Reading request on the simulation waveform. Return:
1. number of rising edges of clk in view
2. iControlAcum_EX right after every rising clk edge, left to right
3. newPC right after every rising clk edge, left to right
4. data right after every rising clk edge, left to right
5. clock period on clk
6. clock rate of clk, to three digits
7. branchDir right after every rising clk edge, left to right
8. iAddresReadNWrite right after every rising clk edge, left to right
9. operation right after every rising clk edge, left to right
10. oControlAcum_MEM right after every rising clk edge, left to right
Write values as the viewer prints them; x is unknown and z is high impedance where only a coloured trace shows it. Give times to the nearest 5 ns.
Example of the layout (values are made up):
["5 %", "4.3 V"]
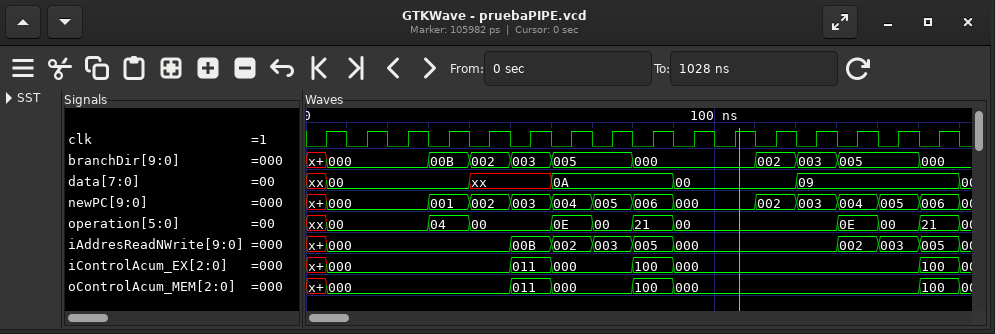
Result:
["16", "000, 000, 000, 000, 000, 011, 000, 000, 100, 000, 000, 000, 000, 000, 000, 100", "000, 000, 000, 001, 002, 003, 004, 005, 006, 000, 000, 002, 003, 004, 005, 006", "00, 00, 00, 00, xx, xx, 0A, 0A, 0A, 00, 00, 00, 09, 09, 09, 09", "10 ns", "100 MHz", "000, 000, 000, 00B, 002, 003, 005, 005, 000, 000, 000, 002, 003, 005, 005, 000", "000, 000, 000, 000, 000, 00B, 002, 003, 005, 000, 000, 000, 000, 002, 003, 005", "00, 00, 00, 04, 00, 00, 0E, 00, 21, 00, 00, 00, 00, 0E, 00, 21", "000, 000, 000, 000, 000, 011, 000, 000, 100, 000, 000, 000, 000, 000, 000, 100"]
